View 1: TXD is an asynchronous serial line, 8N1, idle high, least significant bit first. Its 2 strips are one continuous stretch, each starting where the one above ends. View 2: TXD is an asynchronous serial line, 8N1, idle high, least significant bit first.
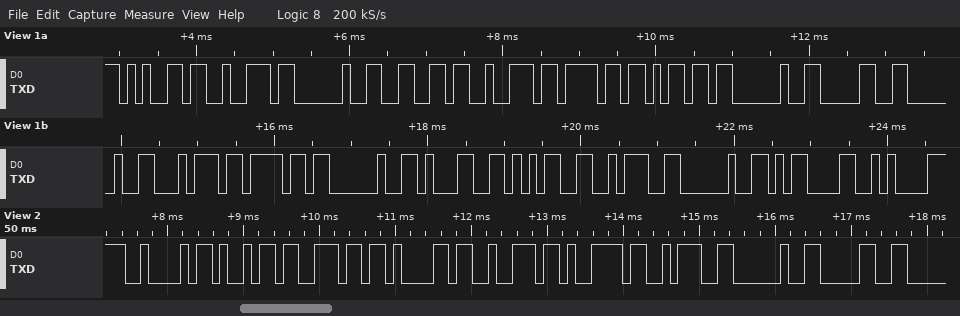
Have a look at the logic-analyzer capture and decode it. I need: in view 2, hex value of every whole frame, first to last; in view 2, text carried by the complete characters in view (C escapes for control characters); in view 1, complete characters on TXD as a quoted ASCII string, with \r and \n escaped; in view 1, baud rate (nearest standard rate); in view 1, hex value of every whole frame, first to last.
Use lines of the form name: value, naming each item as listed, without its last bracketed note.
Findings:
in view 2, hex value of every whole frame, first to last: 0x42 0x69 0x6E 0x61 0x72 0x79 0x3A 0x20 0x30
in view 2, text carried by the complete characters in view: "Binary: 0"
in view 1, complete characters on TXD as a quoted ASCII string, with \r and \n escaped: "er from 0 to 15: \r\n"
in view 1, baud rate: 9600 baud
in view 1, hex value of every whole frame, first to last: 0x65 0x72 0x20 0x66 0x72 0x6F 0x6D 0x20 0x30 0x20 0x74 0x6F 0x20 0x31 0x35 0x3A 0x20 0x0D 0x0A
